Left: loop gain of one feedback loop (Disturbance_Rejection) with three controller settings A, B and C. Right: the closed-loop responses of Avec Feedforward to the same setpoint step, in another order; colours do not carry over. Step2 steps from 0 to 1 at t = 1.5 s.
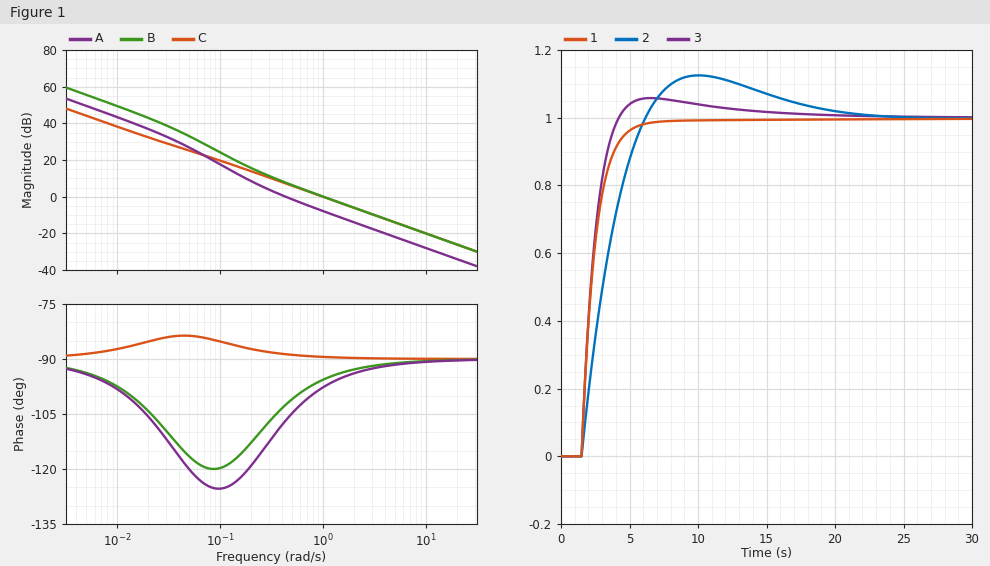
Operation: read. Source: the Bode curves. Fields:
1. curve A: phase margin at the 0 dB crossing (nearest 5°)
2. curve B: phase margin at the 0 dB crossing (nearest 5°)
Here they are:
75°
85°
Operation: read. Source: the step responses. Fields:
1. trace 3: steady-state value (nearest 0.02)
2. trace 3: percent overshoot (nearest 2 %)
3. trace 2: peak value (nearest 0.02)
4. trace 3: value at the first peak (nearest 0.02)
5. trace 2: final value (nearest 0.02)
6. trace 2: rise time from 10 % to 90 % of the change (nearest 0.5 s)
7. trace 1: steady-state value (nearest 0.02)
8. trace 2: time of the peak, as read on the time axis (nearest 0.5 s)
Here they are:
1.00
6 %
1.12
1.06
1.00
3.5 s
1.00
10.0 s
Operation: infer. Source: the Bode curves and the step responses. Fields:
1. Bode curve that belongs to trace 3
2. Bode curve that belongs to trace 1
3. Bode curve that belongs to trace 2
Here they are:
B
C
A
